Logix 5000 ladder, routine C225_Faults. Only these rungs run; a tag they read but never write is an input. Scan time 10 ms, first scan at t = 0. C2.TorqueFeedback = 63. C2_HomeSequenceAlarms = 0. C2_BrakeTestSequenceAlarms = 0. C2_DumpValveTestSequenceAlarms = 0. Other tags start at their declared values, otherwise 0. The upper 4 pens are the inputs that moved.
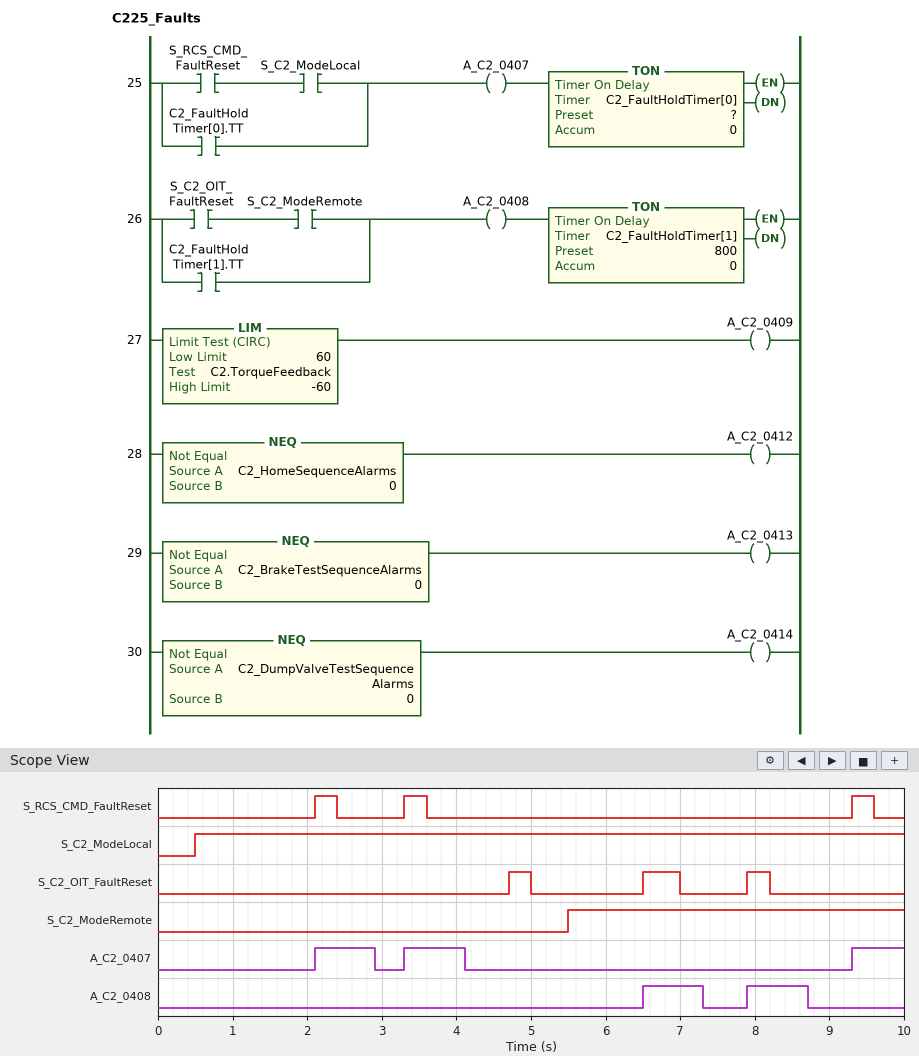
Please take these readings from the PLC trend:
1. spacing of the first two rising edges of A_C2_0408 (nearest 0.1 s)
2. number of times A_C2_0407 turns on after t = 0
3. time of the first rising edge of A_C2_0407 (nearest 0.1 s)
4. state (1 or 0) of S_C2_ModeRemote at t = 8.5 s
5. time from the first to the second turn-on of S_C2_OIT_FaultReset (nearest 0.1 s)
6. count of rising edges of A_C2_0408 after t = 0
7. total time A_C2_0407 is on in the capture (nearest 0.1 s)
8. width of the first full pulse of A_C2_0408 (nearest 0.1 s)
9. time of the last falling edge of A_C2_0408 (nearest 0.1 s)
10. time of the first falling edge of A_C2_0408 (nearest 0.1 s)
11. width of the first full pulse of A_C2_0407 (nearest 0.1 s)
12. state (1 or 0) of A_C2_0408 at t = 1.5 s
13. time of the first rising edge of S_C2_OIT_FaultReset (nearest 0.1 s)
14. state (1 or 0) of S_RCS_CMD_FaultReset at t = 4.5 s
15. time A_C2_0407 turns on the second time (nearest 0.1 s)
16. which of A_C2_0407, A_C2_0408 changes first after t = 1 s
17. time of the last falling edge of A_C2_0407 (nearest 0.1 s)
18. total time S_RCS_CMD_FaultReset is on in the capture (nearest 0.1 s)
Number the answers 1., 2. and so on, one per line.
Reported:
1. 1.4 s
2. 3
3. 2.1 s
4. 1
5. 1.8 s
6. 2
7. 2.3 s
8. 0.8 s
9. 8.7 s
10. 7.3 s
11. 0.8 s
12. 0
13. 4.7 s
14. 0
15. 3.3 s
16. A_C2_0407
17. 4.1 s
18. 0.9 s
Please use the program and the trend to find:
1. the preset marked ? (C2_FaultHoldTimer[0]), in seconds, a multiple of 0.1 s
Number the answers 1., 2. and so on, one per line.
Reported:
1. 0.8 s
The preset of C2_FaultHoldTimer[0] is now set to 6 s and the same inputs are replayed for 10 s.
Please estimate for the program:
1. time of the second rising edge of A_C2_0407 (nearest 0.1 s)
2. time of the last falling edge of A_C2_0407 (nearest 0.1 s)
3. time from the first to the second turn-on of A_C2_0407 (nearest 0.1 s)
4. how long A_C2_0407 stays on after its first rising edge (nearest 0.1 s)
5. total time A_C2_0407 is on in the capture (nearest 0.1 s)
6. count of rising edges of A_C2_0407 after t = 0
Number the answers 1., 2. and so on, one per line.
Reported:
1. 9.3 s
2. 8.1 s
3. 7.2 s
4. 6.0 s
5. 6.7 s
6. 2
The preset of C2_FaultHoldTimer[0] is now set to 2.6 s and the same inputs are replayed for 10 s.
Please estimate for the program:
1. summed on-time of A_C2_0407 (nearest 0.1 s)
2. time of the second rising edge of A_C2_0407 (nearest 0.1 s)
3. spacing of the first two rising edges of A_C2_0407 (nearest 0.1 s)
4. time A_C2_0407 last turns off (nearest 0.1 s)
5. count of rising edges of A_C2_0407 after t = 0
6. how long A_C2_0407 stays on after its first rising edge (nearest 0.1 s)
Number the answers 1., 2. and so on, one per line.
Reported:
1. 3.3 s
2. 9.3 s
3. 7.2 s
4. 4.7 s
5. 2
6. 2.6 s
